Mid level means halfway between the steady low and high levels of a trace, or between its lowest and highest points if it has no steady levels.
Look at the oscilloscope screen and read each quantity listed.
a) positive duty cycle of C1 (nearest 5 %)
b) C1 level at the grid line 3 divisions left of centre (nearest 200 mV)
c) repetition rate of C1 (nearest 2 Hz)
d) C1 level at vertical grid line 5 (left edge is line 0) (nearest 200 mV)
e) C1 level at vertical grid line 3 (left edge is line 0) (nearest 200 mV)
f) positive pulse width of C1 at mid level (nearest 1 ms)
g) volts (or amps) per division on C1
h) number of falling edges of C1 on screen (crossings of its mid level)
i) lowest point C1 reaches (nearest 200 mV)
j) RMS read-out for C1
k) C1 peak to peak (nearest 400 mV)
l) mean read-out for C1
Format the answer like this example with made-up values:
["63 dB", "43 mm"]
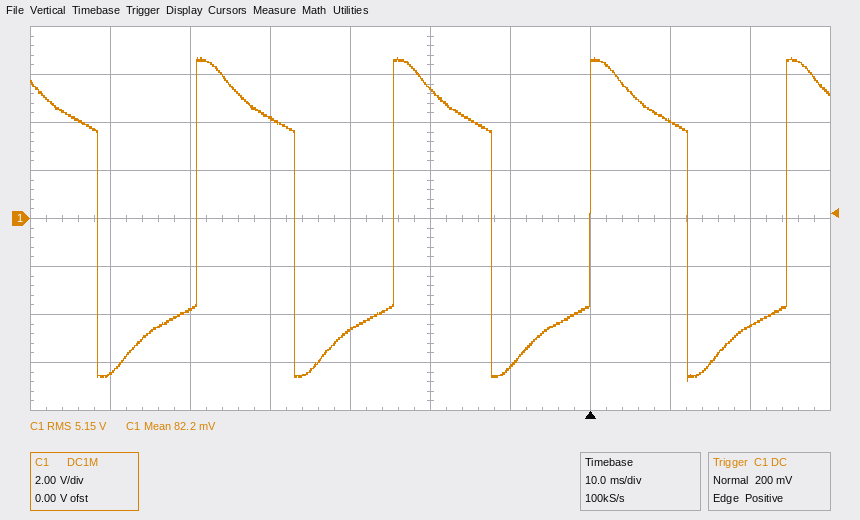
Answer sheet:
["50 %", "-3.8 V", "40 Hz", "5.4 V", "4.2 V", "12 ms", "2 V", "4", "-6.8 V", "5.15 V", "13.6 V", "82.2 mV"]
